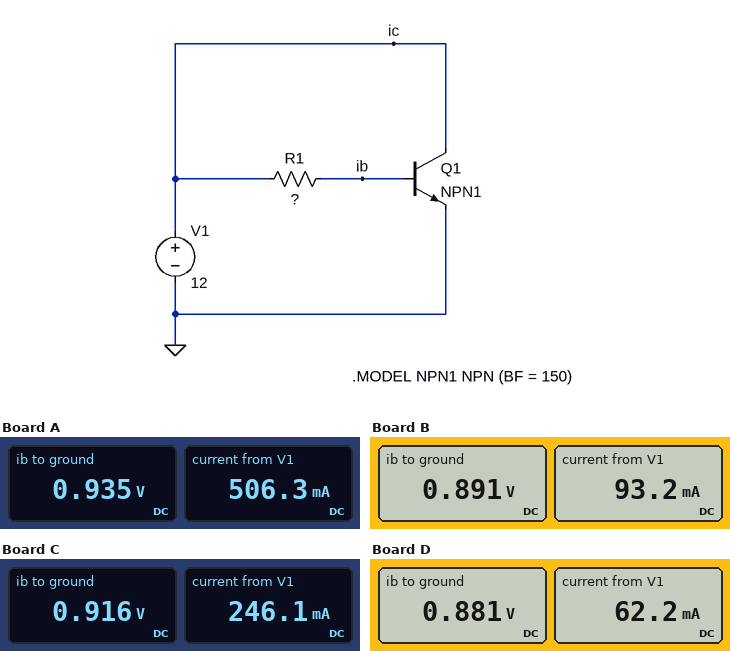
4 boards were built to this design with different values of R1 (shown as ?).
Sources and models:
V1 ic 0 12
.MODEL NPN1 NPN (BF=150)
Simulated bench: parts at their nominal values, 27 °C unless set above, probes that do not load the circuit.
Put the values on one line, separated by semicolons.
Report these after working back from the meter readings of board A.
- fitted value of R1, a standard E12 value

3.3 kΩ
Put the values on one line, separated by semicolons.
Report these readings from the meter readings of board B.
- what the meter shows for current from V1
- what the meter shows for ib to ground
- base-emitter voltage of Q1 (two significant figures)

93.2 mA; 0.891 V; 890 mV
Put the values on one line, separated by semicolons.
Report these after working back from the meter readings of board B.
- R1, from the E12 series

18 kΩ
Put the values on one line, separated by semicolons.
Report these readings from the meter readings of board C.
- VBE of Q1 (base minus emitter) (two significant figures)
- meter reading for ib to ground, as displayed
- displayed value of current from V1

920 mV; 0.916 V; 246.1 mA
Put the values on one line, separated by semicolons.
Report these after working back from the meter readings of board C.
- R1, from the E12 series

6.8 kΩ
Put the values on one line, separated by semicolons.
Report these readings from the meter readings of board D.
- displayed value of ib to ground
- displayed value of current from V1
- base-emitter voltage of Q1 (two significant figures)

0.881 V; 62.2 mA; 880 mV
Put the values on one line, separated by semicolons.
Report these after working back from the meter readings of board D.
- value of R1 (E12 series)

27 kΩ
